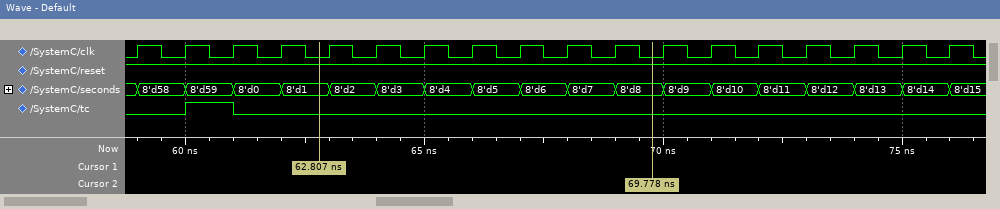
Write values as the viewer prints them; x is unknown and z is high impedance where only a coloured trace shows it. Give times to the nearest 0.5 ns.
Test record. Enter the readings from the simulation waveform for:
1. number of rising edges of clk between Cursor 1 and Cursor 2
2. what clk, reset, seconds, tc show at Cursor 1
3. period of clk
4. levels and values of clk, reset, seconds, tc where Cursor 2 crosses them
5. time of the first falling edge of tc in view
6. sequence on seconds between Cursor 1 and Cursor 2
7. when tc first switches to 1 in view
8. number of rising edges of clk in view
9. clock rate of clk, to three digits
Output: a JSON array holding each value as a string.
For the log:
["7", "clk=0, reset=1, seconds=8'd1, tc=0", "1 ns", "clk=0, reset=1, seconds=8'd8, tc=0", "61 ns", "8'd1, 8'd2, 8'd3, 8'd4, 8'd5, 8'd6, 8'd7, 8'd8", "60 ns", "18", "1.00 GHz"]
